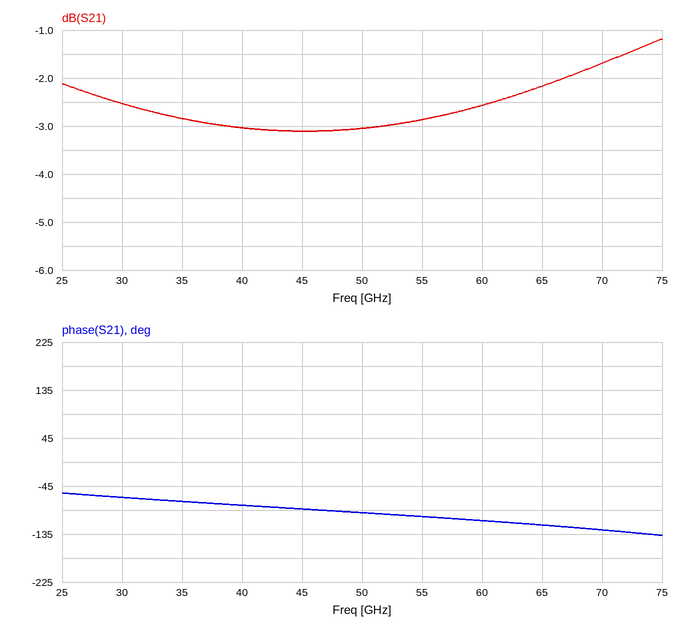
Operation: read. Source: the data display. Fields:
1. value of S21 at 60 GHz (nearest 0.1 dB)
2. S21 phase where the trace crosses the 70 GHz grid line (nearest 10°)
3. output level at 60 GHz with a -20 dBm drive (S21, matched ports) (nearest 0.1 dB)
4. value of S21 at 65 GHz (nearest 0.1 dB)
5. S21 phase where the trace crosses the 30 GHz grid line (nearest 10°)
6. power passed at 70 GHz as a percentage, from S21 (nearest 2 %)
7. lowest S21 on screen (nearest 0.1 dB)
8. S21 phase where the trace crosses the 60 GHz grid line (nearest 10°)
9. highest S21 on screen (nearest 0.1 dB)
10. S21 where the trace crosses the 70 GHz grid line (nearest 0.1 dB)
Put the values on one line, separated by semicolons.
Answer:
-2.6 dB; -130°; -22.6 dBm; -2.2 dB; -70°; 68 %; -3.1 dB; -110°; -1.2 dB; -1.7 dB
